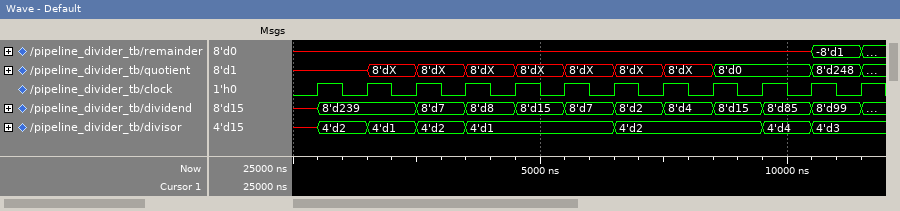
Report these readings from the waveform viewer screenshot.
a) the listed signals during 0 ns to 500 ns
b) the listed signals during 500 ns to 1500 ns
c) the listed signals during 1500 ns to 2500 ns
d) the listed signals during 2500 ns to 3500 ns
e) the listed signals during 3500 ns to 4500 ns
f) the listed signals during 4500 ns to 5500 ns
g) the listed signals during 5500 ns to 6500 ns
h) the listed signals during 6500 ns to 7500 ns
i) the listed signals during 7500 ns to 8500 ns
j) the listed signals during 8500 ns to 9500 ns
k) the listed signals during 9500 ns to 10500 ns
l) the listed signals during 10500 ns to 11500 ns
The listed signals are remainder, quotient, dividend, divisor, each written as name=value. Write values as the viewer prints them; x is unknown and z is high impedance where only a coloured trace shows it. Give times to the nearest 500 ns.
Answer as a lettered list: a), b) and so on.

a) remainder=x, quotient=x, dividend=x, divisor=x
b) remainder=x, quotient=x, dividend=8'd239, divisor=4'd2
c) remainder=x, quotient=8'dX, dividend=8'd239, divisor=4'd1
d) remainder=x, quotient=8'dX, dividend=8'd7, divisor=4'd2
e) remainder=x, quotient=8'dX, dividend=8'd8, divisor=4'd1
f) remainder=x, quotient=8'dX, dividend=8'd15, divisor=4'd1
g) remainder=x, quotient=8'dX, dividend=8'd7, divisor=4'd1
h) remainder=x, quotient=8'dX, dividend=8'd2, divisor=4'd2
i) remainder=x, quotient=8'dX, dividend=8'd4, divisor=4'd2
j) remainder=x, quotient=8'd0, dividend=8'd15, divisor=4'd2
k) remainder=x, quotient=8'd0, dividend=8'd85, divisor=4'd4
l) remainder=-8'd1, quotient=8'd248, dividend=8'd99, divisor=4'd3
